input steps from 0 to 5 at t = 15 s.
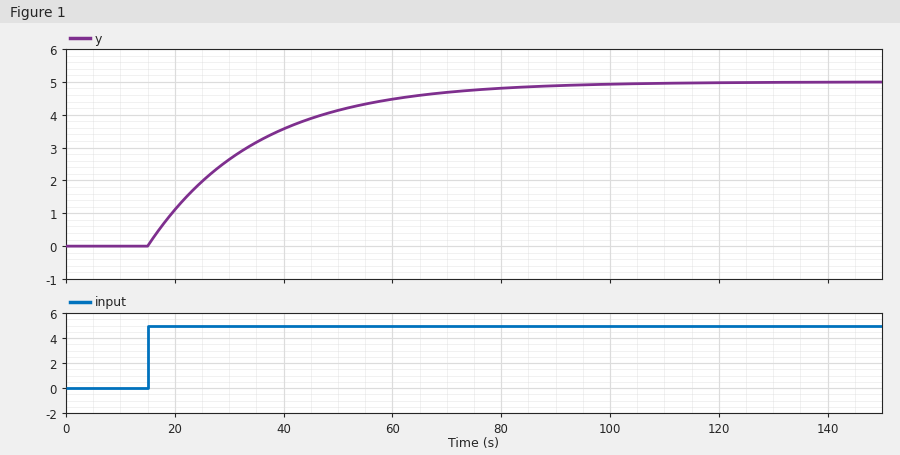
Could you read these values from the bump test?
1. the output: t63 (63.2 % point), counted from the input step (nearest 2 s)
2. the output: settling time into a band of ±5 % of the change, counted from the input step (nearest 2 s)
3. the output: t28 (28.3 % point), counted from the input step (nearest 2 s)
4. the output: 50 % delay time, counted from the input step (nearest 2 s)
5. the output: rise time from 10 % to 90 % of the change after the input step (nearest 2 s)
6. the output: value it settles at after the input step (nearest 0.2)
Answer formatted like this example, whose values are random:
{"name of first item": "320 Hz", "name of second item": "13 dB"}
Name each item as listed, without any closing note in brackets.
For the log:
{"the output: t63 (63.2 % point), counted from the input step": "20 s", "the output: settling time into a band of ±5 % of the change, counted from the input step": "60 s", "the output: t28 (28.3 % point), counted from the input step": "6 s", "the output: 50 % delay time, counted from the input step": "14 s", "the output: rise time from 10 % to 90 % of the change after the input step": "44 s", "the output: value it settles at after the input step": "5.0"}
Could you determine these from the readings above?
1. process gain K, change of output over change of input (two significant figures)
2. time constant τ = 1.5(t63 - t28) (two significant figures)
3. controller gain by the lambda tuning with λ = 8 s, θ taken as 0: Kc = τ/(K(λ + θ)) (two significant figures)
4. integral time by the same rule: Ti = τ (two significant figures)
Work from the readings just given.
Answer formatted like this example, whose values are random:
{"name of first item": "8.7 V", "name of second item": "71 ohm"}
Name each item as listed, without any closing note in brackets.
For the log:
{"process gain K, change of output over change of input": "1.0", "time constant τ = 1.5(t63 - t28)": "21 s", "controller gain by the lambda tuning with λ = 8 s, θ taken as 0: Kc = τ/(K(λ + θ))": "2.6", "integral time by the same rule: Ti = τ": "21 s"}
